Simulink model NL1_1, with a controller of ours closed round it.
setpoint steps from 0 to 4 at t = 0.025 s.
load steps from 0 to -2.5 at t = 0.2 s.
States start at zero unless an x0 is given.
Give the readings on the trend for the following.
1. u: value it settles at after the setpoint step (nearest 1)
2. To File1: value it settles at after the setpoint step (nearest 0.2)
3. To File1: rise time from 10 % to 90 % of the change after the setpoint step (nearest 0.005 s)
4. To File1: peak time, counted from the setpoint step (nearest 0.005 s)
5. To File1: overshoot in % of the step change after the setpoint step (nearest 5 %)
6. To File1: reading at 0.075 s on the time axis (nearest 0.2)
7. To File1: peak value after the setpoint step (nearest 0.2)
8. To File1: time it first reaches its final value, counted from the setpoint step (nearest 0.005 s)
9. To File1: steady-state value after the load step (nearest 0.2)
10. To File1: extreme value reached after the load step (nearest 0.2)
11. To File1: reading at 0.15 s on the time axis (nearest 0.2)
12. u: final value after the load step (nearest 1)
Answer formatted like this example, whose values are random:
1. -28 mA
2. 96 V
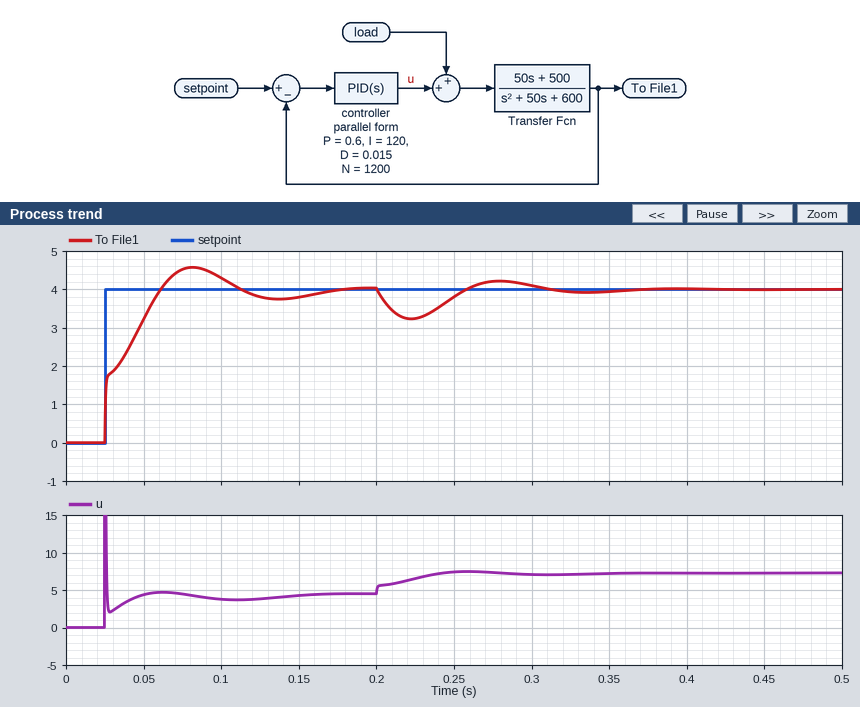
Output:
1. 5
2. 4.0
3. 0.030 s
4. 0.055 s
5. 15 %
6. 4.6
7. 4.6
8. 0.035 s
9. 4.0
10. 3.2
11. 3.8
12. 7
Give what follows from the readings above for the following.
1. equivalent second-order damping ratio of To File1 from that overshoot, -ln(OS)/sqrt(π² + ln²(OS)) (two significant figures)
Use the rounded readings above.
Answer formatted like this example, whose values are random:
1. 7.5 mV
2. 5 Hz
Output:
1. 0.52
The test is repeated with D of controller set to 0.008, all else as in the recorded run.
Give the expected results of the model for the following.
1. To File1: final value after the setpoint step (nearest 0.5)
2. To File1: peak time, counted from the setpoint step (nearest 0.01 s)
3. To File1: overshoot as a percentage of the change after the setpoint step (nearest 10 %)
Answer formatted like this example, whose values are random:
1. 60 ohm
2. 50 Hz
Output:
1. 4.0
2. 0.05 s
3. 20 %
